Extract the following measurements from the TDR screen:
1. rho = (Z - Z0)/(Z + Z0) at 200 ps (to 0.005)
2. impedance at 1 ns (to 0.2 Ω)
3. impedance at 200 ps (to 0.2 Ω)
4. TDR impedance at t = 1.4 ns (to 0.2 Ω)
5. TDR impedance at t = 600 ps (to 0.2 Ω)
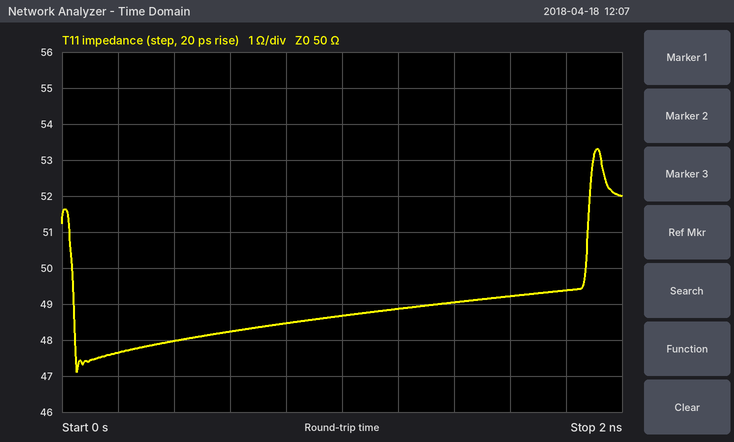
-0.025
48.6 Ω
47.6 Ω
49.0 Ω
48.2 Ω
